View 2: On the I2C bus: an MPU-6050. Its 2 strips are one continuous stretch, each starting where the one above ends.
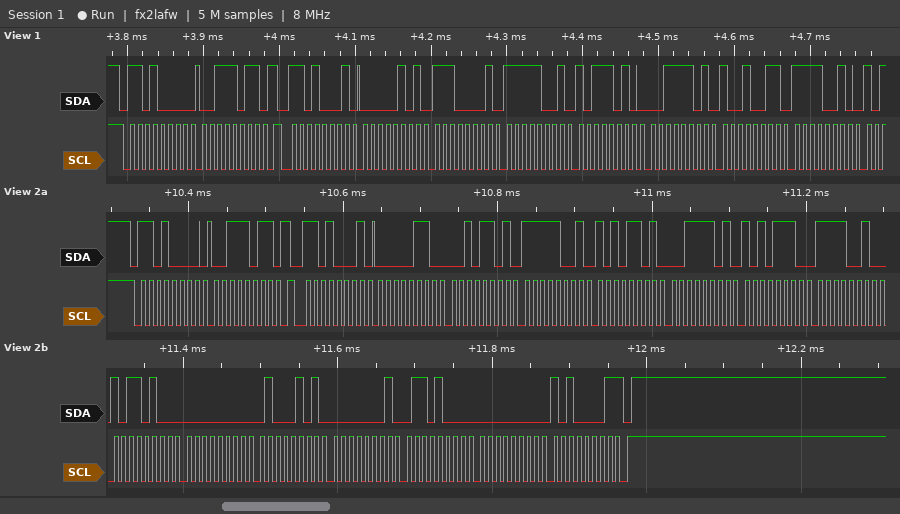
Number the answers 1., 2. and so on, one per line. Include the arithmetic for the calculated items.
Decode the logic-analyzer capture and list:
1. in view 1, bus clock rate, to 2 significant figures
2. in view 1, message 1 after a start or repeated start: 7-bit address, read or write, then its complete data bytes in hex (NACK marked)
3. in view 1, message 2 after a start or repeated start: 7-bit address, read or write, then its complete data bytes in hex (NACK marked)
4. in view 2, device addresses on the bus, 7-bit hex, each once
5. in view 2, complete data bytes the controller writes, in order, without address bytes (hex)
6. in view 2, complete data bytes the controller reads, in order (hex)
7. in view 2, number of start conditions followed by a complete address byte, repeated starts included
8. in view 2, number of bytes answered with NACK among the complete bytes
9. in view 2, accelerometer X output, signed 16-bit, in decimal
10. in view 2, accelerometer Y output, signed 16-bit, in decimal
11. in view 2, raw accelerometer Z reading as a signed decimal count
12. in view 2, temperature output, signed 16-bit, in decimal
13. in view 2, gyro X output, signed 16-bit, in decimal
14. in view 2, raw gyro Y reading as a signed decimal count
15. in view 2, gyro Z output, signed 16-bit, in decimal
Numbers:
1. 100 kHz
2. 0x68 write: 3B
3. 0x68 read: 05 E1 F9 BA 3D 93 F2
4. 0x68
5. 3B
6. 06 2D F9 AD 3D AE F2 B4 00 45 01 68 00 A1
7. 2
8. 1
9. 0x062D = 1581
10. 0xF9AD = -1619
11. 0x3DAE = 15790
12. 0xF2B4 = -3404
13. 0x0045 = 69
14. 0x0168 = 360
15. 0x00A1 = 161
